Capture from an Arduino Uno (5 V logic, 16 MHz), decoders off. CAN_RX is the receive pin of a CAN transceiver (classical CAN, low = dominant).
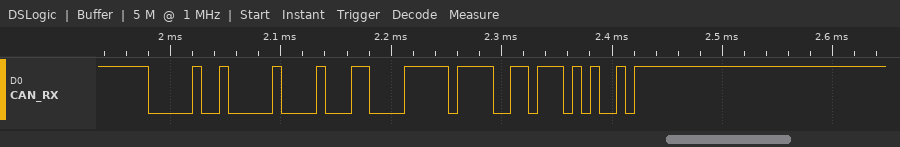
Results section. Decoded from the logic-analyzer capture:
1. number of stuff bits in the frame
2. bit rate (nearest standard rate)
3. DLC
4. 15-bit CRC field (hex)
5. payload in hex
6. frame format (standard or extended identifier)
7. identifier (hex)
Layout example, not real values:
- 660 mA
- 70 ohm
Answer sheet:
- 3
- 125 kbit/s
- 2
- 0x4DD4
- 30 FF
- standard
- 0x010
